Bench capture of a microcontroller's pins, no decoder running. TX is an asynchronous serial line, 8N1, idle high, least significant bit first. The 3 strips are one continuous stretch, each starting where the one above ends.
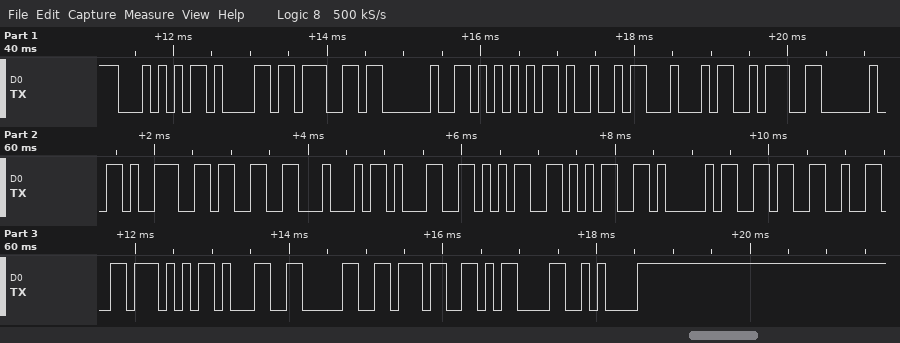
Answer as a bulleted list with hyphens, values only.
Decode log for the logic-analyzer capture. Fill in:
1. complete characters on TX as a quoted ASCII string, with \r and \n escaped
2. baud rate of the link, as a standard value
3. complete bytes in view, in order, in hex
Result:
- "Tag UID: 93D155A62W107\r\n"
- 9600 baud
- 0x54 0x61 0x67 0x20 0x55 0x49 0x44 0x3A 0x20 0x39 0x33 0x44 0x31 0x35 0x35 0x41 0x36 0x32 0x57 0x31 0x30 0x37 0x0D 0x0A
